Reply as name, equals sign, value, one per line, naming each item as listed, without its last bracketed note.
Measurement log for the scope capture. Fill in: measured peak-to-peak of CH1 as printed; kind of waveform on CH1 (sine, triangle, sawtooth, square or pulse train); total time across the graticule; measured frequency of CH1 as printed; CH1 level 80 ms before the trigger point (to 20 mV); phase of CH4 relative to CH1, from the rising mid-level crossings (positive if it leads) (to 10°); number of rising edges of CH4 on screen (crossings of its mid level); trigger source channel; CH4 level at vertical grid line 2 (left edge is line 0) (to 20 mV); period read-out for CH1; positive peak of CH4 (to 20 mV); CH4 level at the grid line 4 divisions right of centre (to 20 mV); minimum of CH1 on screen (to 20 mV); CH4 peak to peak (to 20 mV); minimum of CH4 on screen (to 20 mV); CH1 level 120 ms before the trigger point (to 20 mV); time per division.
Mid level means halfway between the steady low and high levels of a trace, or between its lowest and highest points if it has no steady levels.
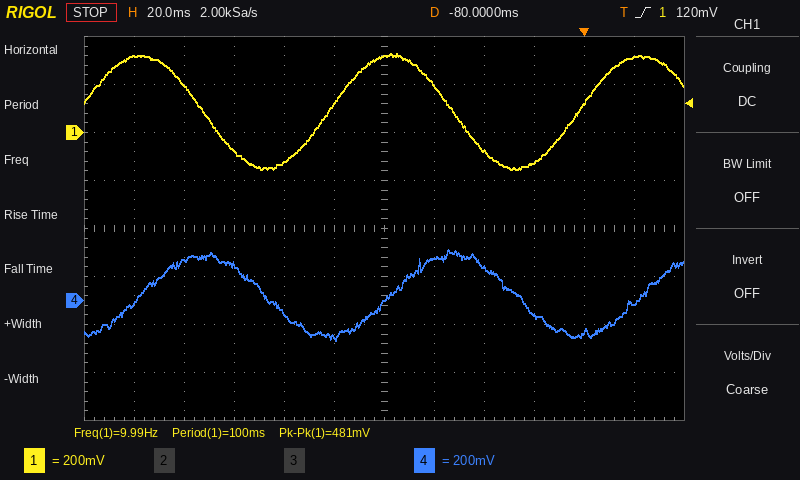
measured peak-to-peak of CH1 as printed = 481 mV
kind of waveform on CH1 = sine
total time across the graticule = 240 ms
measured frequency of CH1 as printed = 9.99 Hz
CH1 level 80 ms before the trigger point = 320 mV
phase of CH4 relative to CH1, from the rising mid-level crossings (positive if it leads) = -90°
number of rising edges of CH4 on screen = 3
trigger source channel = CH1
CH4 level at vertical grid line 2 (left edge is line 0) = 160 mV
period read-out for CH1 = 100 ms
positive peak of CH4 = 220 mV
CH4 level at the grid line 4 divisions right of centre = -140 mV
minimum of CH1 on screen = -160 mV
CH4 peak to peak = 380 mV
minimum of CH4 on screen = -160 mV
CH1 level 120 ms before the trigger point = -120 mV
time per division = 20 ms
